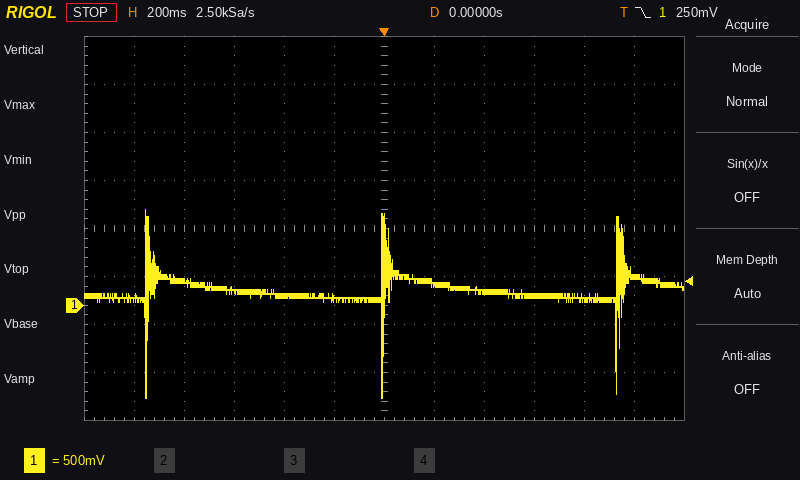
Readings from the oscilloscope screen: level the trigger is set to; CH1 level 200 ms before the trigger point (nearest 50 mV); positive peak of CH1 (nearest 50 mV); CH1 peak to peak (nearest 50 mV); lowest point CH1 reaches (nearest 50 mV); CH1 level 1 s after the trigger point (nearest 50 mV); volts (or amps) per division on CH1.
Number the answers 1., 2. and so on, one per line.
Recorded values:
1. 250 mV
2. 100 mV
3. 1.00 V
4. 1.95 V
5. -950 mV
6. 300 mV
7. 500 mV
